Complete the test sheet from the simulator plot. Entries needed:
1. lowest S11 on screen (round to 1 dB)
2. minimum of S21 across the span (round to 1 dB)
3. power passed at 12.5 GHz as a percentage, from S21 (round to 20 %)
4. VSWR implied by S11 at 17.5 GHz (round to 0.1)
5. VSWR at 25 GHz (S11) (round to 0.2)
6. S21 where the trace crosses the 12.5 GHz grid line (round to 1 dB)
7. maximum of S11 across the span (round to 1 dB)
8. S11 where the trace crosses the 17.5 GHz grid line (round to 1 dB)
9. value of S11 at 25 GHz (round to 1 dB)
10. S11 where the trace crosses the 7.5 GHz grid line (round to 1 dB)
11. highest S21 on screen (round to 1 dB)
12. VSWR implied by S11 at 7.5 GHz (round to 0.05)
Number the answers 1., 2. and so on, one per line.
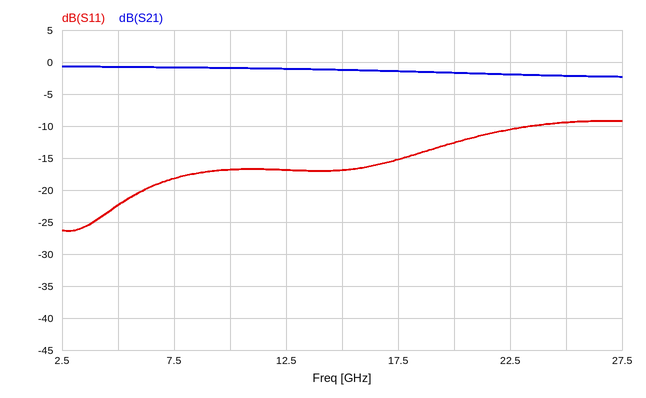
1. -26 dB
2. -2 dB
3. 80 %
4. 1.4
5. 2.0
6. -1 dB
7. -9 dB
8. -15 dB
9. -9 dB
10. -18 dB
11. -1 dB
12. 1.30
